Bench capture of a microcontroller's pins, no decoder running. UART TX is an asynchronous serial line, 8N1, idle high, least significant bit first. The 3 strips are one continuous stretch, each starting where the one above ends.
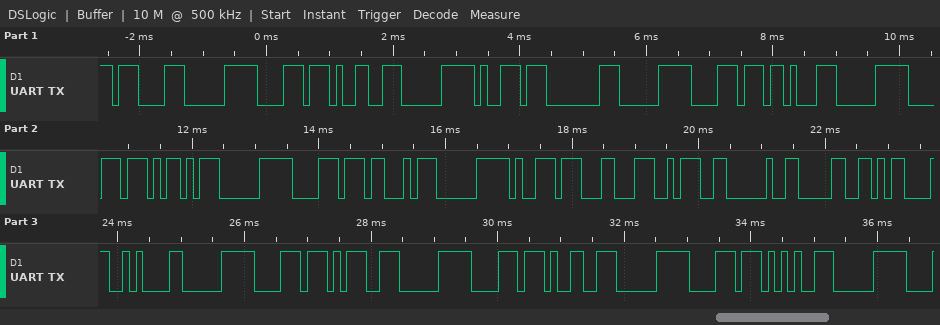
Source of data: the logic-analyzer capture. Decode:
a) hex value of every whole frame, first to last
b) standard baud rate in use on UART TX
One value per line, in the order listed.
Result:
87 E0 B8 99 E0 B9 80 E0 B8 8B E0 B8 AD E0 B8 A3 E0 B9 8C 3A 20 30 0D 0A E0 B8 9D E0 B8 99 E0 B8 95 E0
9600 baud
